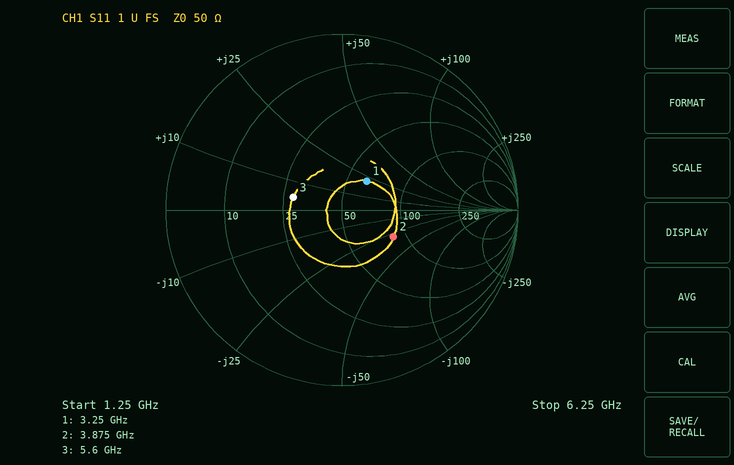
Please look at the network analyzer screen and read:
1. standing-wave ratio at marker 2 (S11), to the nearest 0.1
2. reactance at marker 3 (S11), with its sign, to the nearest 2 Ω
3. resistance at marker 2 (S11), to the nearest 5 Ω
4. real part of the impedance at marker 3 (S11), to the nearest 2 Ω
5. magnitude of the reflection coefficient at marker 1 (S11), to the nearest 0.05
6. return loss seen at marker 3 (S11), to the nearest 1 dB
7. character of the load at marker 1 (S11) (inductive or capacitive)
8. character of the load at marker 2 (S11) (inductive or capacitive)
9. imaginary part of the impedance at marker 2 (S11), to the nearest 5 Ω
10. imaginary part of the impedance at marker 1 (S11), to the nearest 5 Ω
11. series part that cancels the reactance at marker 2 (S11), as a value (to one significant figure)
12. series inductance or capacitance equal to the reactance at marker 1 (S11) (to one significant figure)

2.0
+4 Ω
85 Ω
28 Ω
0.20
11 dB
inductive
capacitive
-30 Ω
+20 Ω
1 nH
1 nH
